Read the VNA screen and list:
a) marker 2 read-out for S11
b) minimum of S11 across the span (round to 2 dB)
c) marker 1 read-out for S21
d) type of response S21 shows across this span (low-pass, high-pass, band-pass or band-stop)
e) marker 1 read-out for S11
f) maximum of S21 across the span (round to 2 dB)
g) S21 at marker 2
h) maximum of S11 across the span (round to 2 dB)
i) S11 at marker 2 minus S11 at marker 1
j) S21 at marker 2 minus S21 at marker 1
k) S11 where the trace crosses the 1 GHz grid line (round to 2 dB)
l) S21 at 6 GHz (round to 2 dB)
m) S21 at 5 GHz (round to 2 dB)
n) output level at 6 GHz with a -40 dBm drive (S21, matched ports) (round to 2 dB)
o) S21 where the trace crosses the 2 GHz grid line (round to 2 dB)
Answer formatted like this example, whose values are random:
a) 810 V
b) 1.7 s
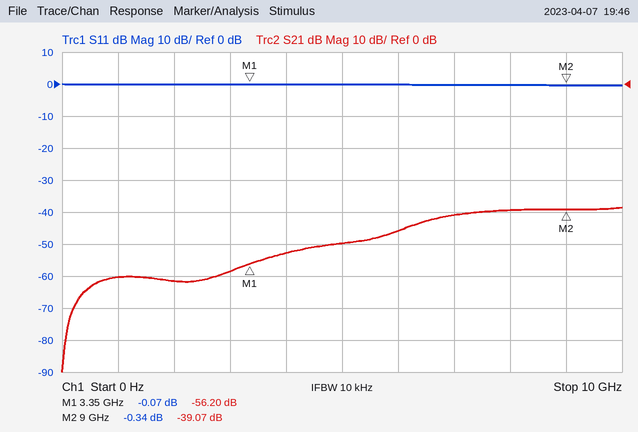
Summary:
a) -0.34 dB
b) 0 dB
c) -56.20 dB
d) high-pass
e) -0.07 dB
f) -38 dB
g) -39.07 dB
h) 0 dB
i) -0.27 dB
j) 17.13 dB
k) 0 dB
l) -46 dB
m) -50 dB
n) -86 dBm
o) -62 dB
